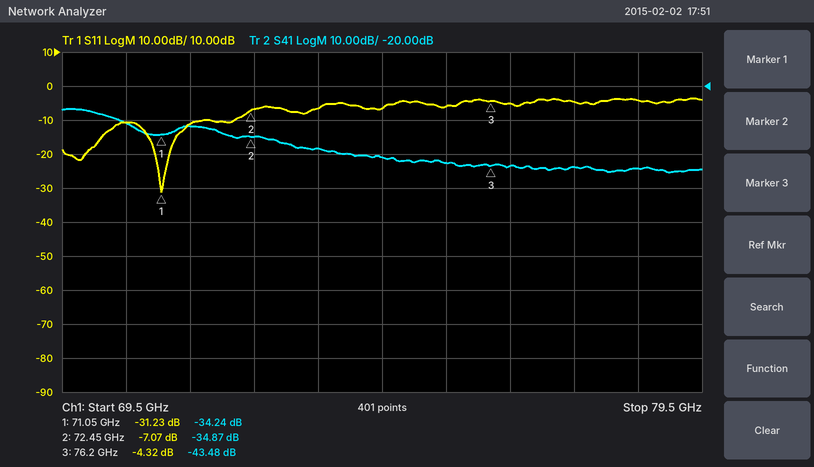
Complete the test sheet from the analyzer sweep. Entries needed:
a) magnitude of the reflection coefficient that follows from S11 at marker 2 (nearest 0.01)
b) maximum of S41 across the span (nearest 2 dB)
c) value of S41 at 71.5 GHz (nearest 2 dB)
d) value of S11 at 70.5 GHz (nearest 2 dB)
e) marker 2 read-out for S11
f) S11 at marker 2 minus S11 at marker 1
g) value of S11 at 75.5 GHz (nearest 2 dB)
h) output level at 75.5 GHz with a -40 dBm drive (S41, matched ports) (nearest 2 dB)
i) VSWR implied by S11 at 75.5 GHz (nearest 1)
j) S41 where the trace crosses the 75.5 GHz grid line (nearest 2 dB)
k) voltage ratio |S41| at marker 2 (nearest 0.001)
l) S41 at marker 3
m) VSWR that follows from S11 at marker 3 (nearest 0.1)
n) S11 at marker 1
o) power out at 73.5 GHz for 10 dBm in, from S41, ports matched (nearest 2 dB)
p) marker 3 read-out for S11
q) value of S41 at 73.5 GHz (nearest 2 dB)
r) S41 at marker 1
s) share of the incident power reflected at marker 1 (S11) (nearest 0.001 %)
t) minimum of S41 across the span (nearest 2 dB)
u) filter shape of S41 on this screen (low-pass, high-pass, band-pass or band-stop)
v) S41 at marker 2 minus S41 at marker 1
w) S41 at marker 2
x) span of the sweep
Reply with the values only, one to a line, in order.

0.44
-26 dB
-32 dB
-10 dB
-7.07 dB
24.16 dB
-6 dB
-82 dBm
3
-42 dB
0.018
-43.48 dB
4.1
-31.23 dB
-28 dBm
-4.32 dB
-38 dB
-34.24 dB
0.075 %
-46 dB
low-pass
-0.63 dB
-34.87 dB
10 GHz
